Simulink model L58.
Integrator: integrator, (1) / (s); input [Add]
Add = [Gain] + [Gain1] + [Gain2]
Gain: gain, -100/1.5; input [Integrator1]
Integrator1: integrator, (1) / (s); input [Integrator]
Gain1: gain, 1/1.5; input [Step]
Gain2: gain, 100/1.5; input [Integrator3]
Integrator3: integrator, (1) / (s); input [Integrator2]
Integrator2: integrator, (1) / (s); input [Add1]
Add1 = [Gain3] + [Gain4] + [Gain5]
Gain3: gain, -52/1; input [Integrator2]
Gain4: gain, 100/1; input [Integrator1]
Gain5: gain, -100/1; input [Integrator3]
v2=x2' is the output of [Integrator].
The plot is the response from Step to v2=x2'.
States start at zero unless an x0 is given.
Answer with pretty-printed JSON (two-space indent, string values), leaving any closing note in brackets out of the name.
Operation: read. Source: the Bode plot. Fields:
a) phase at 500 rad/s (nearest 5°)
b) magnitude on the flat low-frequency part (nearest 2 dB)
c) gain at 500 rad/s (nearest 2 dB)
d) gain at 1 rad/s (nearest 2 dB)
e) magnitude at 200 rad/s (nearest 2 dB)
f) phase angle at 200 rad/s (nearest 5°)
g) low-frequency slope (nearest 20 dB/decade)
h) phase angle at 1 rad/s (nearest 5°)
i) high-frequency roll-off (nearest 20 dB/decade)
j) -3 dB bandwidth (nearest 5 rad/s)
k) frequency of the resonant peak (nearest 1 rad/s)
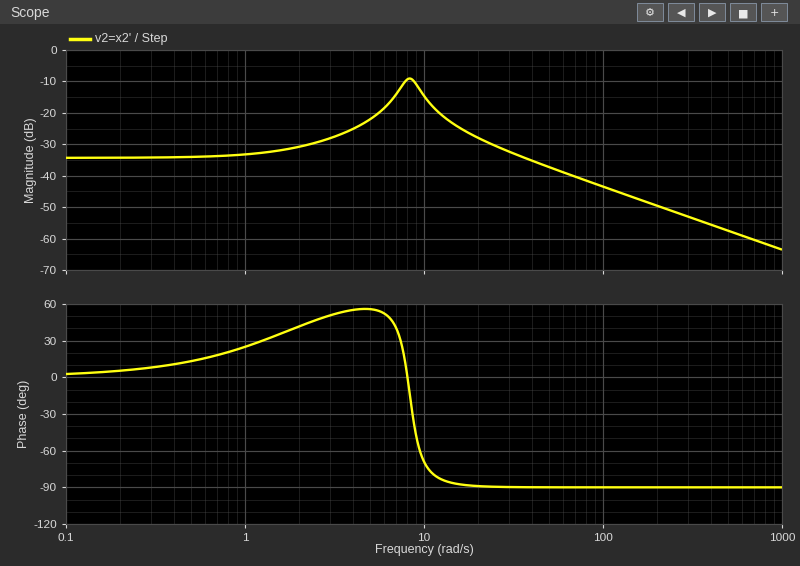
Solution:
{
  "phase at 500 rad/s": "-90°",
  "magnitude on the flat low-frequency part": "-34 dB",
  "gain at 500 rad/s": "-58 dB",
  "gain at 1 rad/s": "-34 dB",
  "magnitude at 200 rad/s": "-50 dB",
  "phase angle at 200 rad/s": "-90°",
  "low-frequency slope": "0 dB/decade",
  "phase angle at 1 rad/s": "25°",
  "high-frequency roll-off": "-20 dB/decade",
  "-3 dB bandwidth": "50 rad/s",
  "frequency of the resonant peak": "8 rad/s"
}
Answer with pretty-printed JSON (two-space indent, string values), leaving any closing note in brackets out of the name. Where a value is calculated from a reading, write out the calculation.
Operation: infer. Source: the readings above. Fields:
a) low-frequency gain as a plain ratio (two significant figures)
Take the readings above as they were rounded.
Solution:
{
  "low-frequency gain as a plain ratio": "10^(-34 / 20) = 0.020"
}
